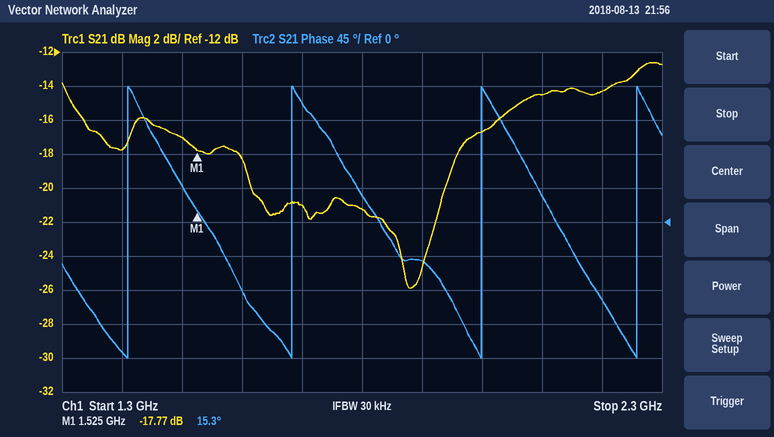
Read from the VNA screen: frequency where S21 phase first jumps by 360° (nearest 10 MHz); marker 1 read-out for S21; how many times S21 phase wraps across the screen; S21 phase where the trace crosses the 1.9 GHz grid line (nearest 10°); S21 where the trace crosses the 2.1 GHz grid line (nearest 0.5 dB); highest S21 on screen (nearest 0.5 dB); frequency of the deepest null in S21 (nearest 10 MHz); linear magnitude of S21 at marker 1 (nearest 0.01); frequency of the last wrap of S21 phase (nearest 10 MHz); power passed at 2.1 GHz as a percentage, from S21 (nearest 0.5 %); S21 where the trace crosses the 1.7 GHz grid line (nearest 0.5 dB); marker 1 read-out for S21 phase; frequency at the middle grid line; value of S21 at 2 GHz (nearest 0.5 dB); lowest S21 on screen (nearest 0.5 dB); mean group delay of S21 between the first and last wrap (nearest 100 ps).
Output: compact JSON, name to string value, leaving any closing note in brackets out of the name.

{"frequency where S21 phase first jumps by 360°": "1.41 GHz", "marker 1 read-out for S21": "-17.77 dB", "how many times S21 phase wraps across the screen": "4", "S21 phase where the trace crosses the 1.9 GHz grid line": "-50°", "S21 where the trace crosses the 2.1 GHz grid line": "-14.5 dB", "highest S21 on screen": "-12.5 dB", "frequency of the deepest null in S21": "1.88 GHz", "linear magnitude of S21 at marker 1": "0.13", "frequency of the last wrap of S21 phase": "2.26 GHz", "power passed at 2.1 GHz as a percentage, from S21": "3.5 %", "S21 where the trace crosses the 1.7 GHz grid line": "-21.0 dB", "marker 1 read-out for S21 phase": "15.3°", "frequency at the middle grid line": "1.8 GHz", "value of S21 at 2 GHz": "-16.5 dB", "lowest S21 on screen": "-26.0 dB", "mean group delay of S21 between the first and last wrap": "3.5 ns"}
